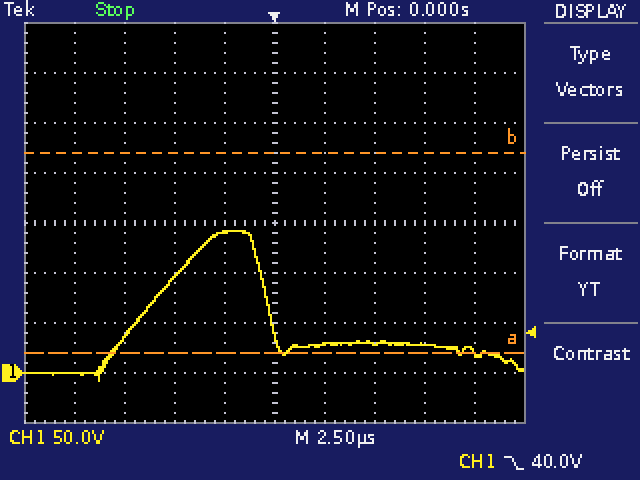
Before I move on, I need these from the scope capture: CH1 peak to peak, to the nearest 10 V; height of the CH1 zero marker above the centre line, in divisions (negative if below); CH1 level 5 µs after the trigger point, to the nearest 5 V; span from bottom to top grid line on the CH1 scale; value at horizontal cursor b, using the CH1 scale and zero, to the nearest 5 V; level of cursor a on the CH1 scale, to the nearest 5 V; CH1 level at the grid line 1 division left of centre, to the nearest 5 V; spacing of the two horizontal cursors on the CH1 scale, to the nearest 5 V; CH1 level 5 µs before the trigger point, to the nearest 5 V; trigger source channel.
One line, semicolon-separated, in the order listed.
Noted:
150 V; -3.0 div; 30 V; 400 V; 220 V; 20 V; 140 V; 200 V; 95 V; CH1
